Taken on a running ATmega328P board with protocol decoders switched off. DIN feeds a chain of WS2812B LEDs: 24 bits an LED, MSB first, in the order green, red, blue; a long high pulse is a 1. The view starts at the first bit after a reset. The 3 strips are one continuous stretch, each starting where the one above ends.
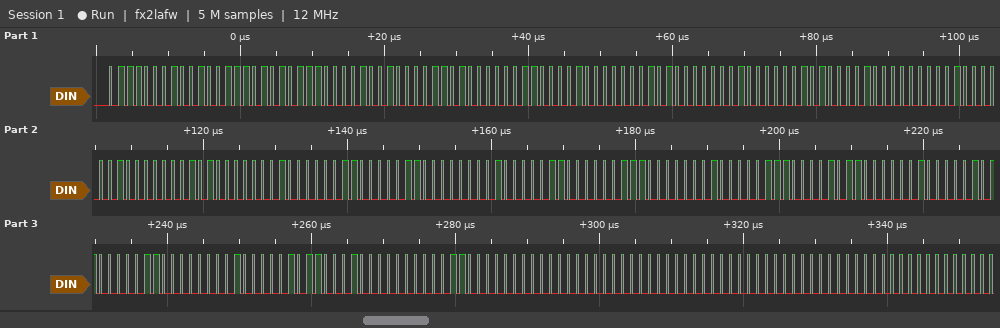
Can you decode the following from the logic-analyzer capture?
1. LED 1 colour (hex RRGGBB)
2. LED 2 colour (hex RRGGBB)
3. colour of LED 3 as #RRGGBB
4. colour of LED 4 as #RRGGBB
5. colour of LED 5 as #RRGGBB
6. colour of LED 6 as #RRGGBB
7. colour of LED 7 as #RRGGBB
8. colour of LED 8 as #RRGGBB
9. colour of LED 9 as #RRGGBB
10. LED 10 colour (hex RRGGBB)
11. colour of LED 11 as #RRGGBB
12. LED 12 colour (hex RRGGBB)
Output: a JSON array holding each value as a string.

["#277157", "#0D0903", "#0A0802", "#080502", "#050401", "#060301", "#070601", "#0B0702", "#0C0A02", "#100B03", "#000000", "#000000"]
